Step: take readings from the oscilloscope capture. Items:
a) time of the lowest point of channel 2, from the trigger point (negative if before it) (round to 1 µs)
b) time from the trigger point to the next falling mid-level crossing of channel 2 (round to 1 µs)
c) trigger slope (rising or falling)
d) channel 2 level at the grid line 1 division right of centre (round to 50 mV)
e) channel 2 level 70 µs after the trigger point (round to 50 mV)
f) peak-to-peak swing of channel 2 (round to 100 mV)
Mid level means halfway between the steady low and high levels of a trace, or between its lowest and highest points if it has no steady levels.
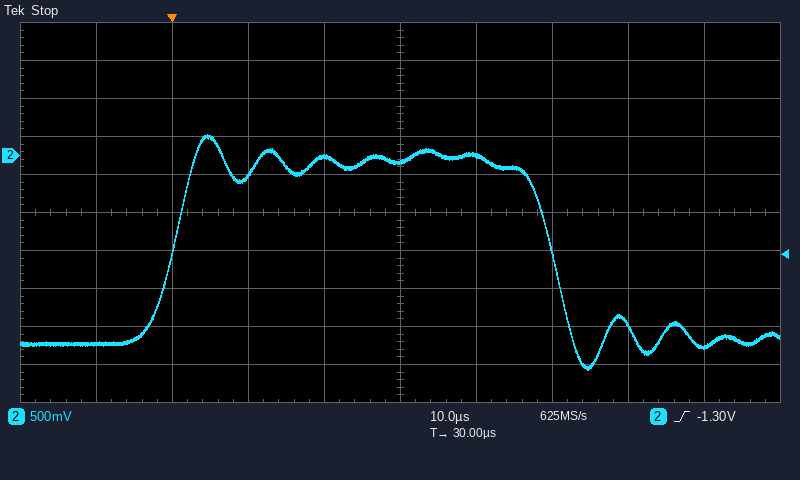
+55 µs
50 µs
rising
0 mV
-2.50 V
3.10 V
